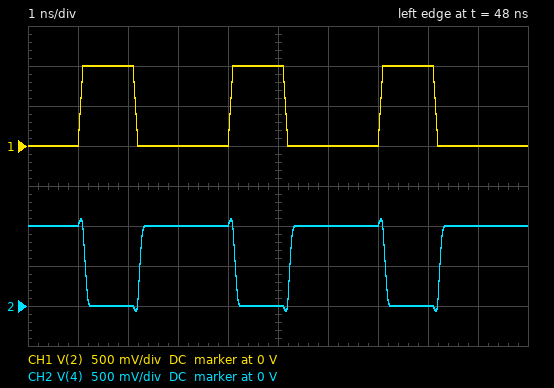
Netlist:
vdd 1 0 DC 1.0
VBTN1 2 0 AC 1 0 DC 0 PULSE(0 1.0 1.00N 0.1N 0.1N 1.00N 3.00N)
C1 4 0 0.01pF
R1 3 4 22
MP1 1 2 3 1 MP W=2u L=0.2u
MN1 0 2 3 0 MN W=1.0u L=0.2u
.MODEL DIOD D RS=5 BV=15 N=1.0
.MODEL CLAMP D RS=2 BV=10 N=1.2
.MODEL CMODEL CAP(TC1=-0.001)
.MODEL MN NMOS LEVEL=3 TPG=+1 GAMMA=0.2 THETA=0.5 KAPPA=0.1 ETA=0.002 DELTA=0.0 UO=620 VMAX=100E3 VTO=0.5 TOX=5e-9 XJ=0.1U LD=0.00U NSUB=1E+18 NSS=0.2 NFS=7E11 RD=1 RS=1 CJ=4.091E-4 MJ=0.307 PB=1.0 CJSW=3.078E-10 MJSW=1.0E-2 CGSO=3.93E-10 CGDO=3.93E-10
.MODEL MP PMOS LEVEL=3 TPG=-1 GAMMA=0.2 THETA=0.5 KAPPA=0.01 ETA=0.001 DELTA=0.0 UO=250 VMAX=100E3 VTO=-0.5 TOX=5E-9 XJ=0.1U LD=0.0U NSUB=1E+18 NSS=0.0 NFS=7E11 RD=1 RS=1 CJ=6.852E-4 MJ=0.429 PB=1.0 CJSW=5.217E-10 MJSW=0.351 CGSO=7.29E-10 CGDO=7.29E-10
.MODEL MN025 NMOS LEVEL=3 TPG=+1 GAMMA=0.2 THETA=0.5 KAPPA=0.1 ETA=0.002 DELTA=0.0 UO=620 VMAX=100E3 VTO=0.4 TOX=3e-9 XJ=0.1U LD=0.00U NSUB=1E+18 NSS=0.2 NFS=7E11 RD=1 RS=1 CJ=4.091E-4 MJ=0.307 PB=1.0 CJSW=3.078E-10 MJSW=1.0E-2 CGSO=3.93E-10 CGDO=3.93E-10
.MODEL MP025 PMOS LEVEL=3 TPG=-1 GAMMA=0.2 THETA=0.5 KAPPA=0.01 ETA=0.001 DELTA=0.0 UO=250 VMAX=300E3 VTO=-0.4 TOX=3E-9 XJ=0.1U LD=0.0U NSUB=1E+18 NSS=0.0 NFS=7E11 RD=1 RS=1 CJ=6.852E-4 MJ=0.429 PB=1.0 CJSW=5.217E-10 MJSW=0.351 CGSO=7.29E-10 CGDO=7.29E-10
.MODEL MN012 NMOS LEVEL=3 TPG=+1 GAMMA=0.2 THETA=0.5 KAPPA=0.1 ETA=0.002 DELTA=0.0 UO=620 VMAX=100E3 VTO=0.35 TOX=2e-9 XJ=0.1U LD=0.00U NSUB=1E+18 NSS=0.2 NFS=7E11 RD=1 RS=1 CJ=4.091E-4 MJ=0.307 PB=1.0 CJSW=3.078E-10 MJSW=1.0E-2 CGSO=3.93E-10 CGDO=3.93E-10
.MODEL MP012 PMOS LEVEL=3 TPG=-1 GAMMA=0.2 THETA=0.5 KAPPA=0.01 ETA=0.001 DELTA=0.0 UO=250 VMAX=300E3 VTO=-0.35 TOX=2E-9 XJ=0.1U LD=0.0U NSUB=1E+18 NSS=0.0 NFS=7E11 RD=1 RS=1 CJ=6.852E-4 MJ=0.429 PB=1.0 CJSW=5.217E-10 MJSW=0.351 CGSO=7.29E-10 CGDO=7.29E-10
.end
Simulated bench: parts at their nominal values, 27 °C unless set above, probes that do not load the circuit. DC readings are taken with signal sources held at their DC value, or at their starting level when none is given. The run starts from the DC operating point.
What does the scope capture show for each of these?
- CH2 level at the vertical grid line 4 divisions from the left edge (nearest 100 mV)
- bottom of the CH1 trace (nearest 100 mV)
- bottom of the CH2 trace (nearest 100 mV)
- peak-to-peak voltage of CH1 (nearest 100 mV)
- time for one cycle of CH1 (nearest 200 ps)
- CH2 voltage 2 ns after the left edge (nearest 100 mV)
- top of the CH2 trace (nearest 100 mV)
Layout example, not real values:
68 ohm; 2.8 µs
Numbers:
1.0 V; 0 V; -100 mV; 1.0 V; 3.0 ns; 0 V; 1.1 V
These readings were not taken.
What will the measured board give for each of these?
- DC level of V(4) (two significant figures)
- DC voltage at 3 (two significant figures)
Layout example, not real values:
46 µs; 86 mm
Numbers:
1.0 V; 1.0 V
